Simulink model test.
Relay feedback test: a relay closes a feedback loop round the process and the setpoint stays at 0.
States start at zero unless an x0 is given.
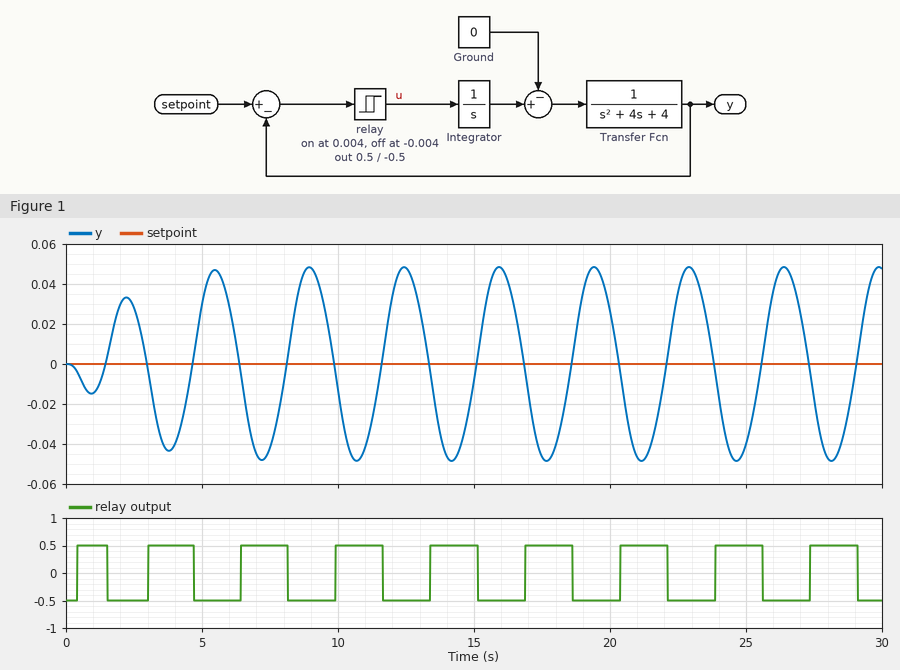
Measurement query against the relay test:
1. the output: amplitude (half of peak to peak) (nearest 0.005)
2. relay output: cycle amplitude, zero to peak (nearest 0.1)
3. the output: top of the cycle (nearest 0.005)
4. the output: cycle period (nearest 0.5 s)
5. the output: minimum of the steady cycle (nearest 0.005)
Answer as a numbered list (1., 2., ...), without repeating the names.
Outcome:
1. 0.050
2. 0.5
3. 0.050
4. 3.5 s
5. -0.050
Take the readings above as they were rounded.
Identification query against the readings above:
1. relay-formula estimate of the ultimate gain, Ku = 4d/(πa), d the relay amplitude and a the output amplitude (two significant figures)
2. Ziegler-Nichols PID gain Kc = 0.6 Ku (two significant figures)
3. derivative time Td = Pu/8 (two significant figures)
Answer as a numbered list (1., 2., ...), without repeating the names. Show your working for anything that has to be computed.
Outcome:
1. 4 × 0.5 / (π × 0.05) = 13
2. 0.6 × 13 = 7.8
3. 3.5 / 8 = 0.44 s
